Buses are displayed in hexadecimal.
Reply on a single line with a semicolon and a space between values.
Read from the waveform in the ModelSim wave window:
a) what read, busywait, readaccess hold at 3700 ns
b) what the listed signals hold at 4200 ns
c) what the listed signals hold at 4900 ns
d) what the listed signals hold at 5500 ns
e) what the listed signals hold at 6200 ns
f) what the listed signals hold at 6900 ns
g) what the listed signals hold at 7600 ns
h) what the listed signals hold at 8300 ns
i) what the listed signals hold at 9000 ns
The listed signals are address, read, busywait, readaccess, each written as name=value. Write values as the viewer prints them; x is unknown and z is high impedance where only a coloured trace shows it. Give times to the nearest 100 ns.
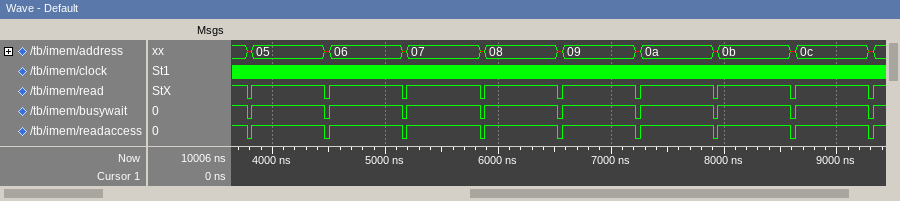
read=1, busywait=1, readaccess=1; address=05, read=1, busywait=1, readaccess=1; address=06, read=1, busywait=1, readaccess=1; address=07, read=1, busywait=1, readaccess=1; address=08, read=1, busywait=1, readaccess=1; address=09, read=1, busywait=1, readaccess=1; address=0a, read=1, busywait=1, readaccess=1; address=0b, read=1, busywait=1, readaccess=1; address=0c, read=1, busywait=1, readaccess=1
